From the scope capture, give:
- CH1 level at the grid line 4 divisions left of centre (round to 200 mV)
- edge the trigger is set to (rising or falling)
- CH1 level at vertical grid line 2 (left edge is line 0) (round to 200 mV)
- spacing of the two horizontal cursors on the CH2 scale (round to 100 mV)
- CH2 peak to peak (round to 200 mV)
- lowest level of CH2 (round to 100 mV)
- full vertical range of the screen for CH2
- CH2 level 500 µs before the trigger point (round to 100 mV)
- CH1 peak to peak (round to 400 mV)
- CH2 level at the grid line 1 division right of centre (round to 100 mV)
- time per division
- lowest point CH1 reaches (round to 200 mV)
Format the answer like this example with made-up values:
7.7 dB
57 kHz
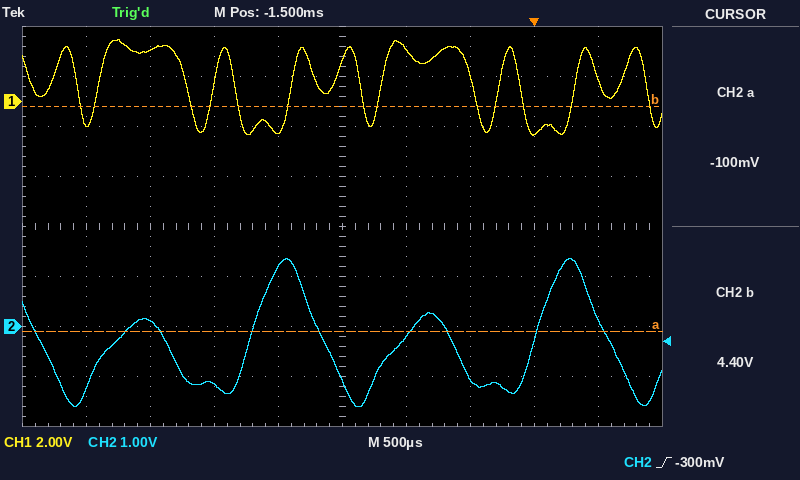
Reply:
-800 mV
rising
2.0 V
4.5 V
3.0 V
-1.6 V
8 V
-1.0 V
4.0 V
-200 mV
500 µs
-1.4 V
